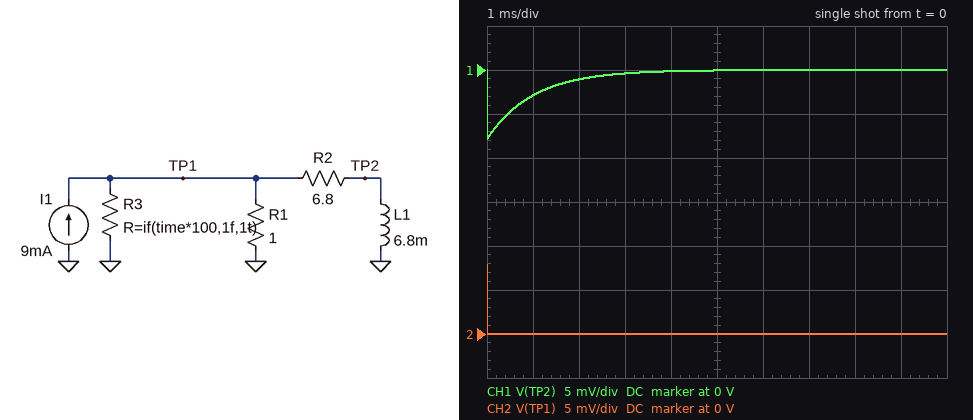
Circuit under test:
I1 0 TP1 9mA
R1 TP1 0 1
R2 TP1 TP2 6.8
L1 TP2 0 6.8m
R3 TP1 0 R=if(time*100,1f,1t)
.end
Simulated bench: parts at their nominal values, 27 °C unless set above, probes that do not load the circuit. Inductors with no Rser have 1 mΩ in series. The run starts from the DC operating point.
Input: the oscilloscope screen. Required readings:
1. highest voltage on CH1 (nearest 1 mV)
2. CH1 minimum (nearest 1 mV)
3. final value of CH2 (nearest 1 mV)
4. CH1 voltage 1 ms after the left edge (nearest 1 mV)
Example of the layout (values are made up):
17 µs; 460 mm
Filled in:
0 V; -8 mV; 0 V; -3 mV
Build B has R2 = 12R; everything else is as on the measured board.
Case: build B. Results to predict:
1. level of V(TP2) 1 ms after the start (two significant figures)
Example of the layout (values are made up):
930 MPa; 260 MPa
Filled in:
-1.4 mV
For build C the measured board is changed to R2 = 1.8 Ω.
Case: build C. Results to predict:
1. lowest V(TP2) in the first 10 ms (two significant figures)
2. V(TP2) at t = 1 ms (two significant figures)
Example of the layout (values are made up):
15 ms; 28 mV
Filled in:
-5.8 mV; -4.4 mV
